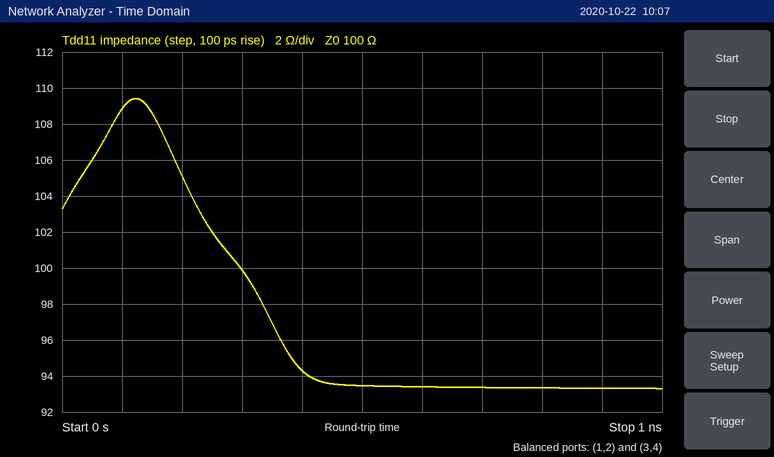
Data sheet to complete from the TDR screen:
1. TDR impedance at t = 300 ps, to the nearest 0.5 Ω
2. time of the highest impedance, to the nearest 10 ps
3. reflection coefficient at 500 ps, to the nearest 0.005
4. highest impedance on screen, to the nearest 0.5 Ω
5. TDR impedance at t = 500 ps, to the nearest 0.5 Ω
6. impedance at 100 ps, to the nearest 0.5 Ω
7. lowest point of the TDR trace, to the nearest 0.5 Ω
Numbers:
100.0 Ω
120 ps
-0.035
109.5 Ω
93.5 Ω
109.0 Ω
93.5 Ω
